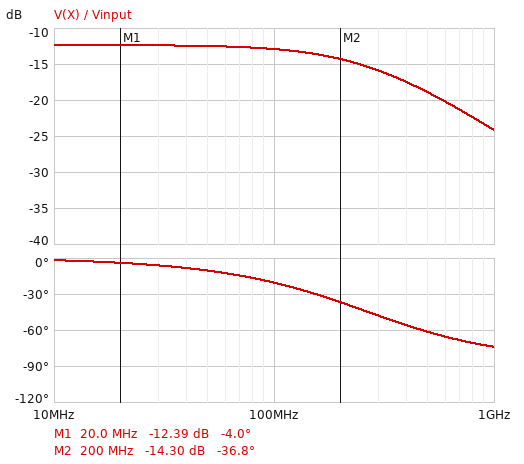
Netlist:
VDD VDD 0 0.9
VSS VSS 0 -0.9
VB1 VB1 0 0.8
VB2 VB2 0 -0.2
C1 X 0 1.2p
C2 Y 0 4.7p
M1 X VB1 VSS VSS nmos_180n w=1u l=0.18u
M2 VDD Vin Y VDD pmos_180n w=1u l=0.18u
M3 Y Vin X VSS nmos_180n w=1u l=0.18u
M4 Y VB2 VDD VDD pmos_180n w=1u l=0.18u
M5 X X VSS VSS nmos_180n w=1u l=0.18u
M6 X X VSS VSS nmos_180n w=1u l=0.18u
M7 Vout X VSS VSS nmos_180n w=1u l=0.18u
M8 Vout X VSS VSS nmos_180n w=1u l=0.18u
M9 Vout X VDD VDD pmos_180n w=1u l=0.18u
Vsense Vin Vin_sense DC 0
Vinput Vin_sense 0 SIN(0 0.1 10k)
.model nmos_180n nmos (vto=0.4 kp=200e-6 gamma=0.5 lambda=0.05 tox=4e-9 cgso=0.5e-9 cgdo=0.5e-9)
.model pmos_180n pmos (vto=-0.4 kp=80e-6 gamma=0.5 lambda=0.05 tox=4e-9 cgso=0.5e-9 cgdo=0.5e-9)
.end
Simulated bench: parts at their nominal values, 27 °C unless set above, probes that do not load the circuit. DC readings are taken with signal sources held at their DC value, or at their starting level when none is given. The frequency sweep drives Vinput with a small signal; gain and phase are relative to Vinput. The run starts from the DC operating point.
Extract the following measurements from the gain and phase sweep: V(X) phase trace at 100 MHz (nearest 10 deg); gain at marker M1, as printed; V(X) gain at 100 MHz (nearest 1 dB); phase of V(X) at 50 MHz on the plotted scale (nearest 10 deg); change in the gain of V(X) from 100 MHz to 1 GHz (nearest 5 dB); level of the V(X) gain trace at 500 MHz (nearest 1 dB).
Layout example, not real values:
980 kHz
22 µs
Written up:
-20 deg
-12.39 dB
-13 dB
-10 deg
-10 dB
-19 dB
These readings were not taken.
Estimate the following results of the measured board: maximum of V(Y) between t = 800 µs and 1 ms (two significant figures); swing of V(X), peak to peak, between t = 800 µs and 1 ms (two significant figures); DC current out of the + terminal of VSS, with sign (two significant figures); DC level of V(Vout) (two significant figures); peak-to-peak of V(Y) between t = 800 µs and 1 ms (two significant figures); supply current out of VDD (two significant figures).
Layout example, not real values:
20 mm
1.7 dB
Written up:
770 mV
47 mV
-99 µA
900 mV
320 mV
99 µA
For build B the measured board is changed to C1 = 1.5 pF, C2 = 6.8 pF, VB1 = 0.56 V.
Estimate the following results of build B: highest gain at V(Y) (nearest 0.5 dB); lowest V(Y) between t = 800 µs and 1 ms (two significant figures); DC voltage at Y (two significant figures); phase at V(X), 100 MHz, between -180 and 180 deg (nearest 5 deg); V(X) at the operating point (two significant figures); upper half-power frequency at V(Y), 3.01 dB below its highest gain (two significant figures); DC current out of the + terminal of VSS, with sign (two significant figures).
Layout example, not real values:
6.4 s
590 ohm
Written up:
1.0 dB
520 mV
690 mV
-30 deg
-820 mV
8.4 MHz
-92 µA
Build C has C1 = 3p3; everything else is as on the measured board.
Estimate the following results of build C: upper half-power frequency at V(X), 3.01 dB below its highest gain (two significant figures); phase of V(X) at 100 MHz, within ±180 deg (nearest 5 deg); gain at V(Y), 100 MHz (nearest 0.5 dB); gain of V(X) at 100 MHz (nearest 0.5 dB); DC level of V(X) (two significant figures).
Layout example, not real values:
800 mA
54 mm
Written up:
99 MHz
-45 deg
-15.0 dB
-15.5 dB
-830 mV
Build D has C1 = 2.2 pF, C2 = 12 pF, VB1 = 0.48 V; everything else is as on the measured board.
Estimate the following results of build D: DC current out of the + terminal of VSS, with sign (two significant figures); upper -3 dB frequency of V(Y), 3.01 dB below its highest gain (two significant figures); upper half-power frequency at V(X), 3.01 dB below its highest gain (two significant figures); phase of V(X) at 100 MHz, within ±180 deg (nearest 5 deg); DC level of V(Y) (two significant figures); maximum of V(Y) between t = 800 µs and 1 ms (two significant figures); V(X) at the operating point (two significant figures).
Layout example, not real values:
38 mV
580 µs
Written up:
-90 µA
4.9 MHz
120 MHz
-40 deg
700 mV
780 mV
-810 mV
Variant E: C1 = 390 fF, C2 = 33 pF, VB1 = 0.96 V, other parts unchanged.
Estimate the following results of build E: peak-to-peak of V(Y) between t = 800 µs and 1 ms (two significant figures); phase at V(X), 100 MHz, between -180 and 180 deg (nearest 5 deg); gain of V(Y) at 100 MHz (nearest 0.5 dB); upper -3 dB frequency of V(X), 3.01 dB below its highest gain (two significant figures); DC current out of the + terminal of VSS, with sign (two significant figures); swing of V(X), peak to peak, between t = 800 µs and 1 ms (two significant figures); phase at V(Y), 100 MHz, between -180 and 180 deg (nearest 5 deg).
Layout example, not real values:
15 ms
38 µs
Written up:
360 mV
-5 deg
-33.0 dB
880 MHz
-100 µA
44 mV
95 deg
